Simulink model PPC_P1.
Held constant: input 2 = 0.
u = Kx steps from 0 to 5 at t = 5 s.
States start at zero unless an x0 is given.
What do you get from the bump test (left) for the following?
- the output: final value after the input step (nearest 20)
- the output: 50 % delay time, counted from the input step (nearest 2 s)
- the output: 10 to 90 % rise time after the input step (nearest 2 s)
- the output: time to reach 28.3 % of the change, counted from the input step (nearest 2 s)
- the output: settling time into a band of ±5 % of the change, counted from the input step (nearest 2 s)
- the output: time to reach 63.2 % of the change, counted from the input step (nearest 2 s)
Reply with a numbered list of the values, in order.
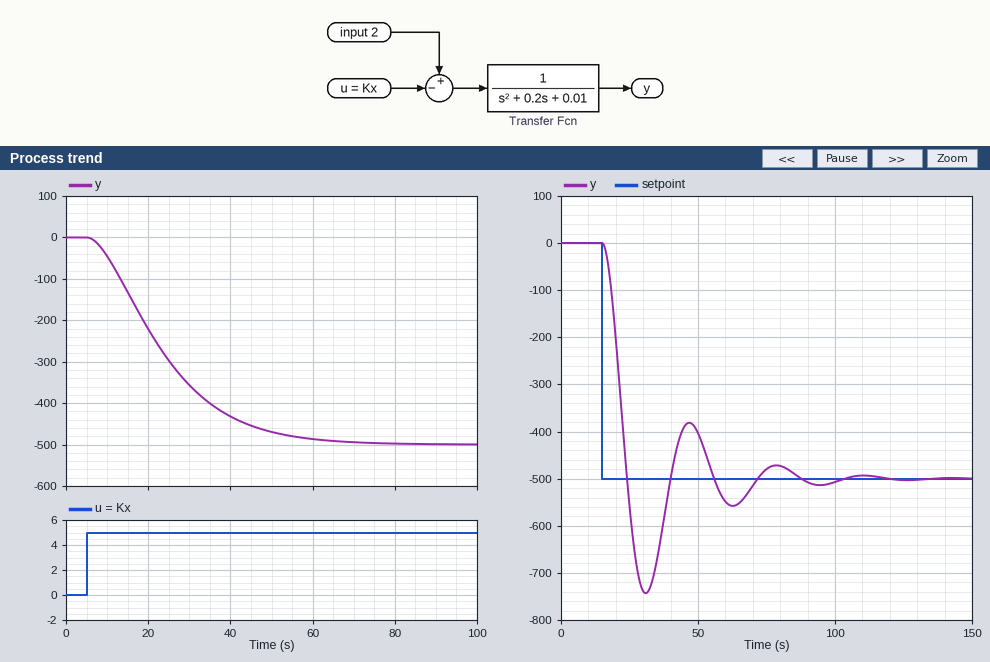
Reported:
1. -500
2. 16 s
3. 34 s
4. 10 s
5. 48 s
6. 22 s
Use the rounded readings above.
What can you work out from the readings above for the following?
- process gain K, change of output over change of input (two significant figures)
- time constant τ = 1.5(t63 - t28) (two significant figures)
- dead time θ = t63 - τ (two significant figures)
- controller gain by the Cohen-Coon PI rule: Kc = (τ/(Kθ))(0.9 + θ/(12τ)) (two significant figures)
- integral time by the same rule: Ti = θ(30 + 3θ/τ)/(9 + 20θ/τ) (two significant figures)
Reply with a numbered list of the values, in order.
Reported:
1. -100
2. 18 s
3. 4.0 s
4. -0.041
5. 9.1 s
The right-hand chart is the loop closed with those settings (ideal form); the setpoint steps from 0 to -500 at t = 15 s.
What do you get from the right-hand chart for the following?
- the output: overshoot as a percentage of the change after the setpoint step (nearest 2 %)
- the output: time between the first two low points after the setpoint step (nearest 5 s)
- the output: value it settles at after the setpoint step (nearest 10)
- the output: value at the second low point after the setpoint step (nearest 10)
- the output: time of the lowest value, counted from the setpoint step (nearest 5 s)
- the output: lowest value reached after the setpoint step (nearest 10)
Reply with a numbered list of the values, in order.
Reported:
1. 48 %
2. 30 s
3. -500
4. -560
5. 15 s
6. -740
